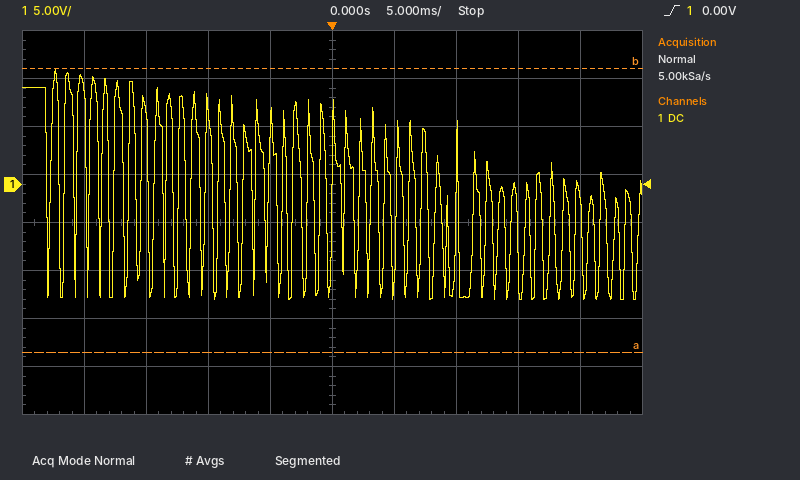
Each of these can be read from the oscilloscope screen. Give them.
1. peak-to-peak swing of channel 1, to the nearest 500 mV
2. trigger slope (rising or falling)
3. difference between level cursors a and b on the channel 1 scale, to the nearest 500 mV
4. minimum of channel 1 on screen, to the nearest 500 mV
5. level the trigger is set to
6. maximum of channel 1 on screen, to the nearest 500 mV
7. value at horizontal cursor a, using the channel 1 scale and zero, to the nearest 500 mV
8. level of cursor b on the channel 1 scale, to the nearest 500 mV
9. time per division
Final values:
24.0 V
rising
29.5 V
-12.0 V
0.00 V
12.0 V
-17.5 V
12.0 V
5 ms
